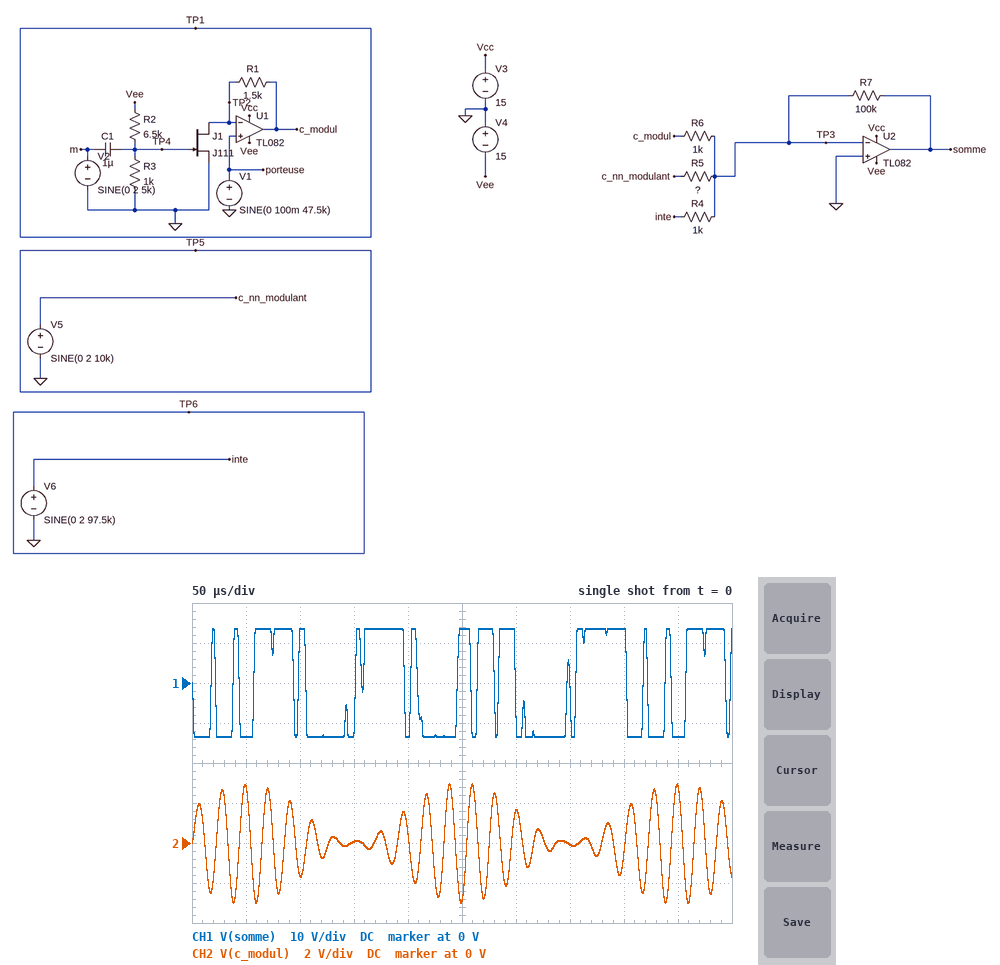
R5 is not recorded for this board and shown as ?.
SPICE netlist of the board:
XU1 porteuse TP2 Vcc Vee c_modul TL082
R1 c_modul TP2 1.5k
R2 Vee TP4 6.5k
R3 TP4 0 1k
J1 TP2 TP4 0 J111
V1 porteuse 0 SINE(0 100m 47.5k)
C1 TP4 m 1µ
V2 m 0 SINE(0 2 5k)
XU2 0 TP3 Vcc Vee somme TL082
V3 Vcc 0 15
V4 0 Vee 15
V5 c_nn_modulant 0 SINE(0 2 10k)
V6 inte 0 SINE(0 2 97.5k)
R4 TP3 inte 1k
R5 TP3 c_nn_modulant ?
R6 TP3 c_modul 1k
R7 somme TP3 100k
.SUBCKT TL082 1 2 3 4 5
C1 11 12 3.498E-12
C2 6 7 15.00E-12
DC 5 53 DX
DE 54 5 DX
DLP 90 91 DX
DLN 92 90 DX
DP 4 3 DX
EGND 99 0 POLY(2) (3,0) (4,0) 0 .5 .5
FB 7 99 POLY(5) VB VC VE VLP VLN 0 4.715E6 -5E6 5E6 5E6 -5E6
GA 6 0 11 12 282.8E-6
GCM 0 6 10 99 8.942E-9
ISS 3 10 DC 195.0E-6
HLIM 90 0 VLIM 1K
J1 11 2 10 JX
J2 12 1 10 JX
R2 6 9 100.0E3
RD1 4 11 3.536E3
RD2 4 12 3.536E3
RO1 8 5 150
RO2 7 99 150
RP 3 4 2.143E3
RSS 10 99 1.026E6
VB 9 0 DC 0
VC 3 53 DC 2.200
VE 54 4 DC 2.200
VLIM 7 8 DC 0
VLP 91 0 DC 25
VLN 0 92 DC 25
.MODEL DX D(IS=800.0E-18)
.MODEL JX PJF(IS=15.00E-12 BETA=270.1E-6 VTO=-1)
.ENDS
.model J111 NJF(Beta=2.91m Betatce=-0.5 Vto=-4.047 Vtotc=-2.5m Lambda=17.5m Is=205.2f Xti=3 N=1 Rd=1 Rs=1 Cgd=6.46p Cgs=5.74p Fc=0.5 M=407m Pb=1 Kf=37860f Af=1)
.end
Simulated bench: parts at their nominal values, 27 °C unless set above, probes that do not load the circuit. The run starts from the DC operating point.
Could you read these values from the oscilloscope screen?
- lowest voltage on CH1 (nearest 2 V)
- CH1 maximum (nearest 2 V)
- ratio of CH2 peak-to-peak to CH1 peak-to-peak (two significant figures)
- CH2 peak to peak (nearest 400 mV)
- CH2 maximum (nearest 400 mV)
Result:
-14 V
14 V
0.22
6.0 V
2.8 V
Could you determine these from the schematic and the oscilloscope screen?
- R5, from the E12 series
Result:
820 Ω
